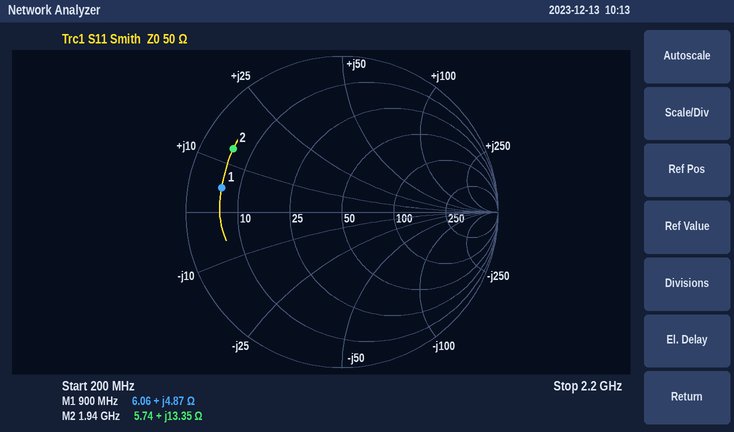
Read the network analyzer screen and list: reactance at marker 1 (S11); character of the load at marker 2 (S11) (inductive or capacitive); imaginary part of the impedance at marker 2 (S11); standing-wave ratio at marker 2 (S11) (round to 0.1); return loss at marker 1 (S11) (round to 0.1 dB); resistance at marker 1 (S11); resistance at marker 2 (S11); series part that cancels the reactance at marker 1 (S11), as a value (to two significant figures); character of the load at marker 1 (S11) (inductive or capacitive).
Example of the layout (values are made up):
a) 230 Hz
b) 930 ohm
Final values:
a) +4.87 Ω
b) inductive
c) +13.35 Ω
d) 9.3
e) 2.1 dB
f) 6.06 Ω
g) 5.74 Ω
h) 36 pF
i) inductive
